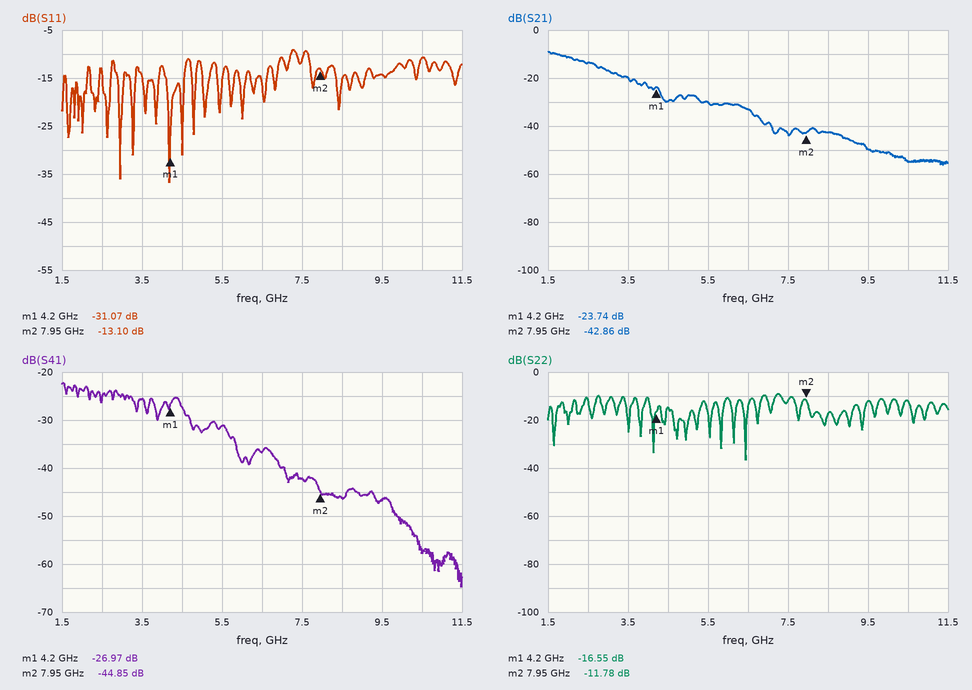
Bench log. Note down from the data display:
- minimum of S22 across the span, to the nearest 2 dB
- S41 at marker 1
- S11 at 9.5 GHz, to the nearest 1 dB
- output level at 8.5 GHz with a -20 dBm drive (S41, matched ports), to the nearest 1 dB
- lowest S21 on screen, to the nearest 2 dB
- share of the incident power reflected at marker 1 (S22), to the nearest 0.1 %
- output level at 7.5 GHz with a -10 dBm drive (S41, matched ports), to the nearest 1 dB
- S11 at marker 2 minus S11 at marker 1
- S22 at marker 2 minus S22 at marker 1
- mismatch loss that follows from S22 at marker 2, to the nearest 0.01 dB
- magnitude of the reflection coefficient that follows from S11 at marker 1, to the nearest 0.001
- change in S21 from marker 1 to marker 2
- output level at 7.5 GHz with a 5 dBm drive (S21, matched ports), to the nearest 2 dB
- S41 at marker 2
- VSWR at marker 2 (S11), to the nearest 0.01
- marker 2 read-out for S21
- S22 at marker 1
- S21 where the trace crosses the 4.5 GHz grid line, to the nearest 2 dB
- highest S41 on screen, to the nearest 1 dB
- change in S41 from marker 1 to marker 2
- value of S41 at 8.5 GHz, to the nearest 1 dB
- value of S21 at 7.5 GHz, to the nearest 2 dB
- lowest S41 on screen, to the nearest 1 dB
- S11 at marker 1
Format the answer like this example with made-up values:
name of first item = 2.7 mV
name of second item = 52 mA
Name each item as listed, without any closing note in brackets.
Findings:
minimum of S22 across the span, to the nearest 2 dB = -36 dB
S41 at marker 1 = -26.97 dB
S11 at 9.5 GHz, to the nearest 1 dB = -14 dB
output level at 8.5 GHz with a -20 dBm drive (S41, matched ports), to the nearest 1 dB = -66 dBm
lowest S21 on screen, to the nearest 2 dB = -56 dB
share of the incident power reflected at marker 1 (S22), to the nearest 0.1 % = 2.2 %
output level at 7.5 GHz with a -10 dBm drive (S41, matched ports), to the nearest 1 dB = -52 dBm
S11 at marker 2 minus S11 at marker 1 = 17.97 dB
S22 at marker 2 minus S22 at marker 1 = 4.77 dB
mismatch loss that follows from S22 at marker 2, to the nearest 0.01 dB = 0.30 dB
magnitude of the reflection coefficient that follows from S11 at marker 1, to the nearest 0.001 = 0.028
change in S21 from marker 1 to marker 2 = -19.12 dB
output level at 7.5 GHz with a 5 dBm drive (S21, matched ports), to the nearest 2 dB = -38 dBm
S41 at marker 2 = -44.85 dB
VSWR at marker 2 (S11), to the nearest 0.01 = 1.57
marker 2 read-out for S21 = -42.86 dB
S22 at marker 1 = -16.55 dB
S21 where the trace crosses the 4.5 GHz grid line, to the nearest 2 dB = -30 dB
highest S41 on screen, to the nearest 1 dB = -22 dB
change in S41 from marker 1 to marker 2 = -17.88 dB
value of S41 at 8.5 GHz, to the nearest 1 dB = -46 dB
value of S21 at 7.5 GHz, to the nearest 2 dB = -44 dB
lowest S41 on screen, to the nearest 1 dB = -65 dB
S11 at marker 1 = -31.07 dB
